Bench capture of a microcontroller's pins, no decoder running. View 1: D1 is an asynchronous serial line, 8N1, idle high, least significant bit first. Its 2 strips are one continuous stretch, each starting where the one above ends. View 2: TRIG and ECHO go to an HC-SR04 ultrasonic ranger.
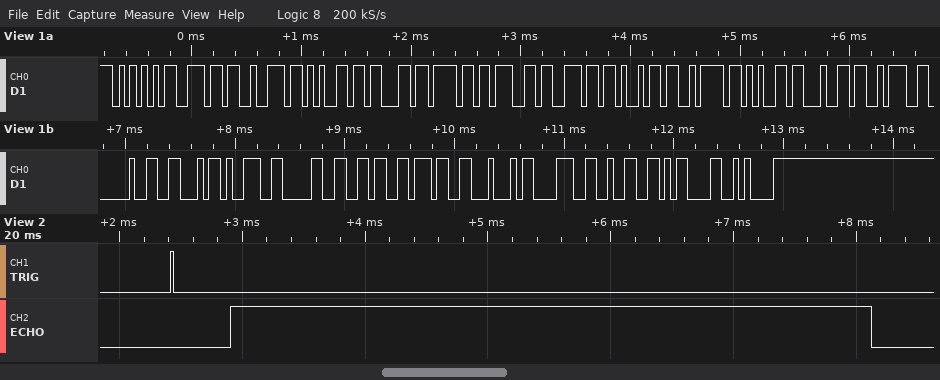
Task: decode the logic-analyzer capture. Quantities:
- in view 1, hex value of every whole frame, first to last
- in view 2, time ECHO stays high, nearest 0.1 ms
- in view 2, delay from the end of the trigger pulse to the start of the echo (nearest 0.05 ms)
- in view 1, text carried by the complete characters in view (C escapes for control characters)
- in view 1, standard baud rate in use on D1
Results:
55 6E 72 65 63 6F 67 6E 69 7A 65 64 3A 20 46 39 30 36 37 44 38 32 0D 0A
5.2 ms
0.45 ms
"Unrecognized: F9067D82\r\n"
19200 baud
